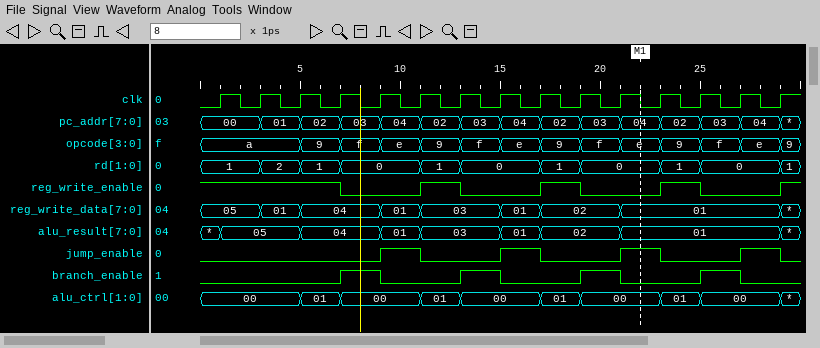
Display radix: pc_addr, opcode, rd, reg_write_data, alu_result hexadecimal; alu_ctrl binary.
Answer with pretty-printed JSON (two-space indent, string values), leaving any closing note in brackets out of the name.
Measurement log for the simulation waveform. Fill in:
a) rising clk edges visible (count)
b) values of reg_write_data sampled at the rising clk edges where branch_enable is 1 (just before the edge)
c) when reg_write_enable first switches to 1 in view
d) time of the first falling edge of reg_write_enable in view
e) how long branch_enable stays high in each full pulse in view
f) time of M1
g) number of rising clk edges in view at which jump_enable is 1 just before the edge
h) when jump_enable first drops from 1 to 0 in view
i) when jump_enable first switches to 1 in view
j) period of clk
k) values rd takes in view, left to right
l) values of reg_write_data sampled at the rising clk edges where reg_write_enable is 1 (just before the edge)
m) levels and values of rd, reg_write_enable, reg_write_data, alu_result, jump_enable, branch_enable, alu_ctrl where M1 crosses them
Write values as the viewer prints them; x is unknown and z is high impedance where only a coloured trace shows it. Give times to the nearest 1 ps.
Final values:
{
  "rising clk edges visible": "15",
  "values of reg_write_data sampled at the rising clk edges where branch_enable is 1": "04, 03, 02, 01",
  "when reg_write_enable first switches to 1 in view": "11 ps",
  "time of the first falling edge of reg_write_enable in view": "7 ps",
  "how long branch_enable stays high in each full pulse in view": "2 ps, 2 ps, 2 ps, 2 ps",
  "time of M1": "22 ps",
  "number of rising clk edges in view at which jump_enable is 1 just before the edge": "4",
  "when jump_enable first drops from 1 to 0 in view": "11 ps",
  "when jump_enable first switches to 1 in view": "9 ps",
  "period of clk": "2 ps",
  "values rd takes in view, left to right": "1, 2, 1, 0, 1, 0, 1, 0, 1, 0, 1",
  "values of reg_write_data sampled at the rising clk edges where reg_write_enable is 1": "05, 05, 01, 04, 03, 02, 01",
  "levels and values of rd, reg_write_enable, reg_write_data, alu_result, jump_enable, branch_enable, alu_ctrl where M1 crosses them": "rd=0, reg_write_enable=0, reg_write_data=01, alu_result=01, jump_enable=1, branch_enable=0, alu_ctrl=00"
}
